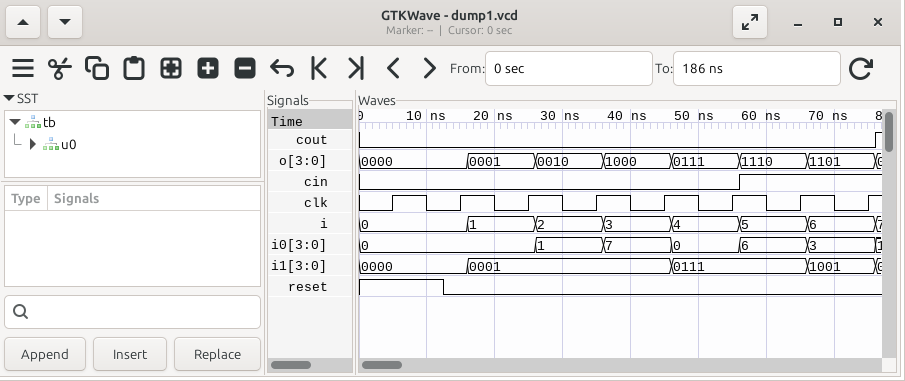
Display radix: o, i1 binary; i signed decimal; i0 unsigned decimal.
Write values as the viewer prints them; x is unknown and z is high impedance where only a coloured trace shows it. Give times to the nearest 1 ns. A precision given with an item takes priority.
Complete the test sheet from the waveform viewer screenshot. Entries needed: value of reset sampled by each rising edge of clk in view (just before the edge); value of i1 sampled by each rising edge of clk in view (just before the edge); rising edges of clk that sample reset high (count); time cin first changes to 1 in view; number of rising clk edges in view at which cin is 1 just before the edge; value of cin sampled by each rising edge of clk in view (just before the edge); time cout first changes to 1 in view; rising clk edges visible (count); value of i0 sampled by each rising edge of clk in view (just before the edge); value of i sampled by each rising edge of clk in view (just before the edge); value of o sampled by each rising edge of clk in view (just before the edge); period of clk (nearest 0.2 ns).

1 0 0 0 0 0 0 0
0000, 0000, 0001, 0001, 0001, 0111, 0111, 1001
1
56 ns
2
0 0 0 0 0 0 1 1
76 ns
8
0, 0, 0, 1, 7, 0, 6, 3
0, 0, 1, 2, 3, 4, 5, 6
0000, 0000, 0001, 0010, 1000, 0111, 1110, 1101
10 ns
